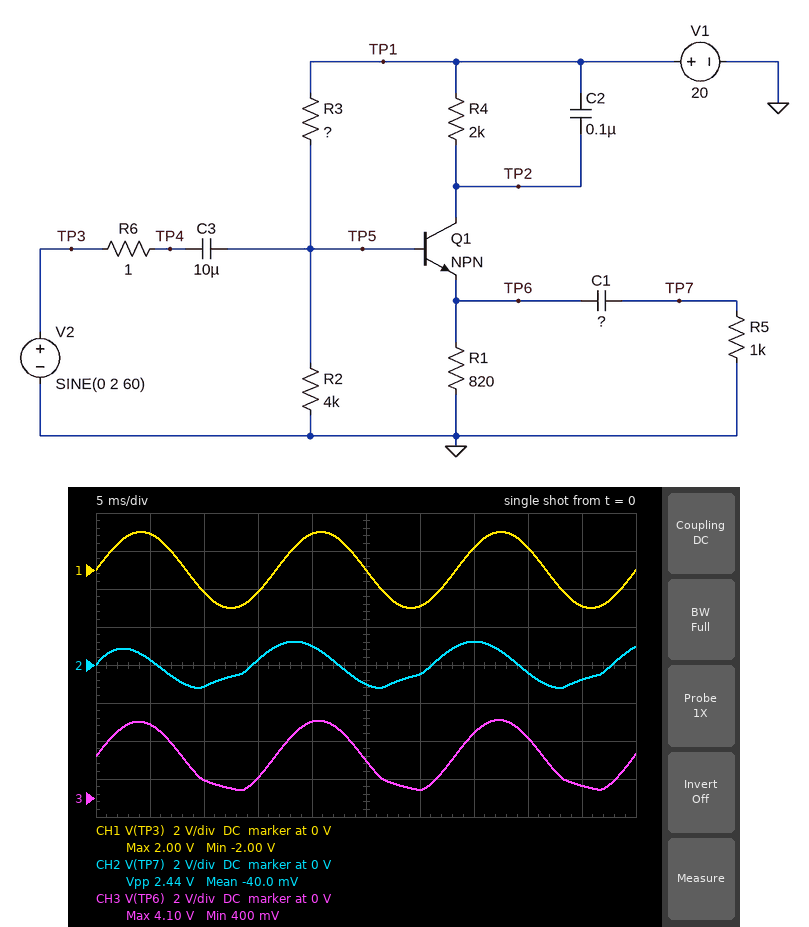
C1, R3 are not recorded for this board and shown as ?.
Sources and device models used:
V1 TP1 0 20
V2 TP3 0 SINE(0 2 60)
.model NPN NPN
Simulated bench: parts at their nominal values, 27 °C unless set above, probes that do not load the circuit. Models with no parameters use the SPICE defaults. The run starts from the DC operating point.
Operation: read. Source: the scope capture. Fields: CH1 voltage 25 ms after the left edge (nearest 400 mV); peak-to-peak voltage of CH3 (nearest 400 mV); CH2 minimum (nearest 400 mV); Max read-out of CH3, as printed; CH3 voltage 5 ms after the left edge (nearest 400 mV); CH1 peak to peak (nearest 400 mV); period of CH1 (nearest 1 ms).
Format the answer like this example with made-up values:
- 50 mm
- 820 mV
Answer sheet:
- 0 V
- 3.6 V
- -1.2 V
- 4.10 V
- 4.0 V
- 4.0 V
- 17 ms
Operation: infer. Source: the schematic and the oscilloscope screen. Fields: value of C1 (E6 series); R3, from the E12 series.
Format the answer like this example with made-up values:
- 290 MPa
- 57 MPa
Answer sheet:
- 2.2 µF
- 22 kΩ
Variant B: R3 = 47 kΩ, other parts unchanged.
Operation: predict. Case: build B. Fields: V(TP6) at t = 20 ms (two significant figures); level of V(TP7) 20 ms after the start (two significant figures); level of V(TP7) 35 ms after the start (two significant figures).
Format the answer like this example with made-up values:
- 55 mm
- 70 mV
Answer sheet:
- 2.6 V
- 890 mV
- 1.0 V
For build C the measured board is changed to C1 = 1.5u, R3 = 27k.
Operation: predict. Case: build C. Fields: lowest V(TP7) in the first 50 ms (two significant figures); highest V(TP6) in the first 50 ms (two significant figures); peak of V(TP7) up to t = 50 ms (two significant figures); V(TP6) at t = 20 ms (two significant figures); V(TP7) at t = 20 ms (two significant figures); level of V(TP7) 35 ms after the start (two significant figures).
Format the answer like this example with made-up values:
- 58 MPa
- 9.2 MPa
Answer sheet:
- -930 mV
- 3.6 V
- 940 mV
- 3.5 V
- 660 mV
- 930 mV
